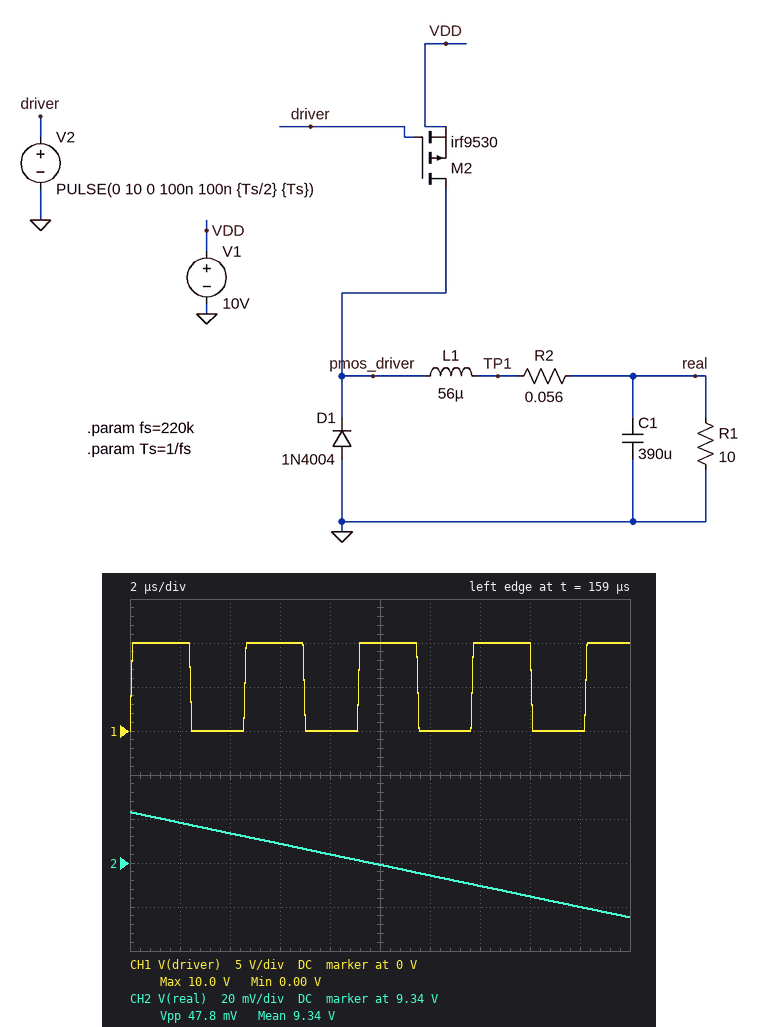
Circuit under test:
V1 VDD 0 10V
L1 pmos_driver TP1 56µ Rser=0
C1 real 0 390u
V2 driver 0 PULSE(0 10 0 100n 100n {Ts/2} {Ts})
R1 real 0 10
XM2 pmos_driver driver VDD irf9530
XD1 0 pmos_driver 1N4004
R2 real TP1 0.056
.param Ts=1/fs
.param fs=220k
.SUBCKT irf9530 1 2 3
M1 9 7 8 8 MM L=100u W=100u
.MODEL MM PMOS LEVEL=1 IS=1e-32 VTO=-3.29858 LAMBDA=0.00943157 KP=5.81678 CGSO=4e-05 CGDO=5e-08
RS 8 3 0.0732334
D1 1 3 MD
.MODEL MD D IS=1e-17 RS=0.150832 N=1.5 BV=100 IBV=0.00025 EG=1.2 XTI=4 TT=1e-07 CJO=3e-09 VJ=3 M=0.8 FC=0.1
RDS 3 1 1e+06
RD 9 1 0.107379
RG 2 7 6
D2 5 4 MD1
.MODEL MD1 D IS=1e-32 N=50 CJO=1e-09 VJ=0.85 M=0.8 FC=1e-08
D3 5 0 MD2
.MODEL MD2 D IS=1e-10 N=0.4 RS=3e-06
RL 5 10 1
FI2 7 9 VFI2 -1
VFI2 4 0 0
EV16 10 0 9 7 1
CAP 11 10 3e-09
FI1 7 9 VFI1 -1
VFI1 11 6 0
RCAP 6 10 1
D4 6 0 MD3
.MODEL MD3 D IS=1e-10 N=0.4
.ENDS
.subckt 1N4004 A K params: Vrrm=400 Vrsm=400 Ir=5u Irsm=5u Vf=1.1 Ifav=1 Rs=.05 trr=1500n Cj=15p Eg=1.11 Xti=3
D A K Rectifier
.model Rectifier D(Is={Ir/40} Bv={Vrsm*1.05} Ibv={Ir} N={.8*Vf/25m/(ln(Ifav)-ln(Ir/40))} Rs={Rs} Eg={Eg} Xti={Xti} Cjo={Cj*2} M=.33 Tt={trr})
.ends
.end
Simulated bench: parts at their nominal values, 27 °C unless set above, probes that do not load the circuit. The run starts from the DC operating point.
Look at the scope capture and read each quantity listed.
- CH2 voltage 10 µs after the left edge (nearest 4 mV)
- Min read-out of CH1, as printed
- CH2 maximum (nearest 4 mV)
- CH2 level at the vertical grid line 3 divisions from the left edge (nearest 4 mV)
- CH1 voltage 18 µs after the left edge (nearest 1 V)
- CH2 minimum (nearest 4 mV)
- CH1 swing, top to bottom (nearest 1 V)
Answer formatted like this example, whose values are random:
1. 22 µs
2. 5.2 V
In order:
1. 9.340 V
2. 0.00 V
3. 9.364 V
4. 9.348 V
5. 0 V
6. 9.316 V
7. 10 V
